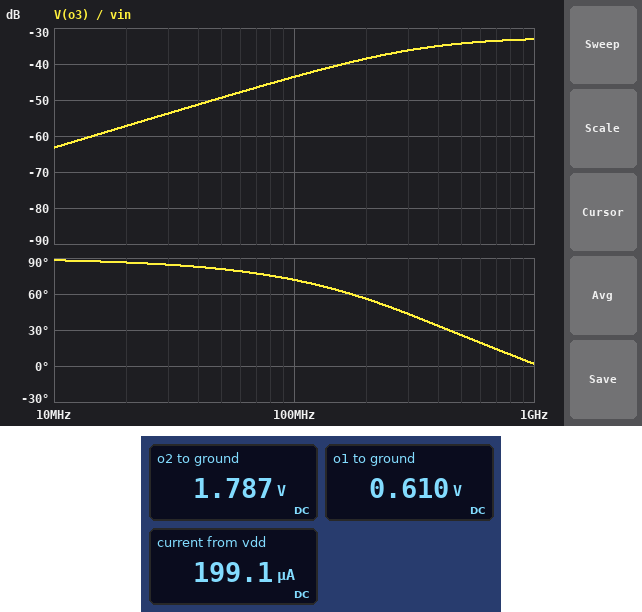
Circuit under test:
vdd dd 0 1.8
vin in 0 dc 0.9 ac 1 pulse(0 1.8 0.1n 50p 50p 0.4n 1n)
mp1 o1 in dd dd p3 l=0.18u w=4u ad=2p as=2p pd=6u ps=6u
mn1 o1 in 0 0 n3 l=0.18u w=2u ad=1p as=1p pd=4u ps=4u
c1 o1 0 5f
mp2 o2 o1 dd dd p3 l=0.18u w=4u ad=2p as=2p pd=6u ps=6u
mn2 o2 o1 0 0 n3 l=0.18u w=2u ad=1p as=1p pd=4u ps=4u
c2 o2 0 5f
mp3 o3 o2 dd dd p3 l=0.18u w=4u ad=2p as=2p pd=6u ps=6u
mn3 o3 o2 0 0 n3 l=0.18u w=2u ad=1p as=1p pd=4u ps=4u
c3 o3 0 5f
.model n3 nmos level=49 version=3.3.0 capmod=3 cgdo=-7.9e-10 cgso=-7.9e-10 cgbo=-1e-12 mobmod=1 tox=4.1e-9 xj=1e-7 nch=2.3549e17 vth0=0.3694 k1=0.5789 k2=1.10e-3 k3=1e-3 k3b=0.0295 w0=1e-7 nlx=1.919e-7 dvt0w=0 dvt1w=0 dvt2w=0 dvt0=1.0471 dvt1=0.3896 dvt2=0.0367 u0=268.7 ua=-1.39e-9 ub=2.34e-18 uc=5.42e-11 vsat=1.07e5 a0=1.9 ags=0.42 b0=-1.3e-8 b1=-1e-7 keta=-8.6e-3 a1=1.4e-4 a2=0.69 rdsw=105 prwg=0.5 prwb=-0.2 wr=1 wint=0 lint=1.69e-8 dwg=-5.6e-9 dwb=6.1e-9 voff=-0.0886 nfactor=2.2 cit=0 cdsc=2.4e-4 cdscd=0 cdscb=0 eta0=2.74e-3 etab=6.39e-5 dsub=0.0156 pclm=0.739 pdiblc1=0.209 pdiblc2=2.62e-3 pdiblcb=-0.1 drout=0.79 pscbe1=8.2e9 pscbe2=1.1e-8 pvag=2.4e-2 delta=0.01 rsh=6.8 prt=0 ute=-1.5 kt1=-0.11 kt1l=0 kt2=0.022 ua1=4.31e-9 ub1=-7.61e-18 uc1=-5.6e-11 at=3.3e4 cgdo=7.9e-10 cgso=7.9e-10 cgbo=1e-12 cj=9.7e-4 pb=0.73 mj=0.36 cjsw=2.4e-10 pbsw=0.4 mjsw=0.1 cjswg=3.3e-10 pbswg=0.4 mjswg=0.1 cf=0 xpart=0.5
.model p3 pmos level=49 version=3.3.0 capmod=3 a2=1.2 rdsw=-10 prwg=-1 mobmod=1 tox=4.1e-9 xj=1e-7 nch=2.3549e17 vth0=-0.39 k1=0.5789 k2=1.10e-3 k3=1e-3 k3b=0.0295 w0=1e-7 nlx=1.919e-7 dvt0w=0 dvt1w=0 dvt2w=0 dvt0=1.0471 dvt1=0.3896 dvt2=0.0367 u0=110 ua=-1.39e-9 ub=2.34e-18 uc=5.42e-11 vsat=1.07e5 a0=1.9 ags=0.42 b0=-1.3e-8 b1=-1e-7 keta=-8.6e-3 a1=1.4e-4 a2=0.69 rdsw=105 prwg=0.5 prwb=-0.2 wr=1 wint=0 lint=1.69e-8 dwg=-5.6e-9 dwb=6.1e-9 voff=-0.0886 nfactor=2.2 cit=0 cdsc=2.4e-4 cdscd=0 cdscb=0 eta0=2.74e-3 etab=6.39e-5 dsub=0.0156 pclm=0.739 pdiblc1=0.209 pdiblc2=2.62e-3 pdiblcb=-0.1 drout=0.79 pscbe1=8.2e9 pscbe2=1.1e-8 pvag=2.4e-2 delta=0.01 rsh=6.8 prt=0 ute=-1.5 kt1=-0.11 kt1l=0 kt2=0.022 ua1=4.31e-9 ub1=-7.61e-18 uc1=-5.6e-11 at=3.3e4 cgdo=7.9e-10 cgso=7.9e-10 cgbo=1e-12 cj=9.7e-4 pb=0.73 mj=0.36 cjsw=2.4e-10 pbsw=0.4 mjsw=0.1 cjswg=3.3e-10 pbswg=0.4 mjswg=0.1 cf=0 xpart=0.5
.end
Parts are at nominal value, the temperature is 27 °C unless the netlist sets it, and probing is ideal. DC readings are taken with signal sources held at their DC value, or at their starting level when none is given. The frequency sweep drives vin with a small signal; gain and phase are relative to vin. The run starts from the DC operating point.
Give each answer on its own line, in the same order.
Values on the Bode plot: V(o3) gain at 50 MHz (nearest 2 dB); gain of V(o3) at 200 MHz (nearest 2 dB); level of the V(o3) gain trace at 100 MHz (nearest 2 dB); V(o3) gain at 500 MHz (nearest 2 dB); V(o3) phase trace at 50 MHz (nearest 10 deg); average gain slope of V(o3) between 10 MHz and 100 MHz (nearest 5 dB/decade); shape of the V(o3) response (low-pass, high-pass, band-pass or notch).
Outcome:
-50 dB
-38 dB
-44 dB
-34 dB
80 deg
20 dB/decade
high-pass
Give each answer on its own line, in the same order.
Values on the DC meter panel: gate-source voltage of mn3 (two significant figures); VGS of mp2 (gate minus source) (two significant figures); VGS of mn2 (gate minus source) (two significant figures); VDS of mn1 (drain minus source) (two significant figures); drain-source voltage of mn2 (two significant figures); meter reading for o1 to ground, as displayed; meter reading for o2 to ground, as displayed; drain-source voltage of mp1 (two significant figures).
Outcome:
1.8 V
-1.2 V
610 mV
610 mV
1.8 V
0.610 V
1.787 V
-1.2 V
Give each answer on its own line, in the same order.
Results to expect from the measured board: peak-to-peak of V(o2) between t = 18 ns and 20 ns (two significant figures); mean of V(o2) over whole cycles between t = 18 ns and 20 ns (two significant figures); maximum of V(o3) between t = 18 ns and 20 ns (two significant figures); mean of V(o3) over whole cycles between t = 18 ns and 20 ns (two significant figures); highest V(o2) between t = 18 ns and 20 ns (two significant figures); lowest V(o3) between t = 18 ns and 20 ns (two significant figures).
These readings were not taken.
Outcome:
2.0 V
810 mV
1.9 V
1.0 V
1.9 V
-84 mV
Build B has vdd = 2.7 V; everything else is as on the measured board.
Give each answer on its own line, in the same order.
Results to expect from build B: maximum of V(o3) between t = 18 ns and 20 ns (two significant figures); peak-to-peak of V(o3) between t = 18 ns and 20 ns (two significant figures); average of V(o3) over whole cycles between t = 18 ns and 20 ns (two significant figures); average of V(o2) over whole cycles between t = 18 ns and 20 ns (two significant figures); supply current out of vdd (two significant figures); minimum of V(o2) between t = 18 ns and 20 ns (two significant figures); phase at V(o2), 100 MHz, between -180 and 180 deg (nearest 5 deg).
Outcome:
2.8 V
2.9 V
1.6 V
1.1 V
240 µA
-55 mV
-90 deg
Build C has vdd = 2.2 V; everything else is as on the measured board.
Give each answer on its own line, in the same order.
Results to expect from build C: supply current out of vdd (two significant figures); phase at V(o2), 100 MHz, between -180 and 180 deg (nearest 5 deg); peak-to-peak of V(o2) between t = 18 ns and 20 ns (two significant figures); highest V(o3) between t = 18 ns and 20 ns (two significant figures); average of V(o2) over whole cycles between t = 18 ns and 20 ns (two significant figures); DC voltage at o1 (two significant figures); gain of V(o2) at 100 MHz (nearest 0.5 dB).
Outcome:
220 µA
-90 deg
2.4 V
2.3 V
950 mV
2.1 V
-60.5 dB
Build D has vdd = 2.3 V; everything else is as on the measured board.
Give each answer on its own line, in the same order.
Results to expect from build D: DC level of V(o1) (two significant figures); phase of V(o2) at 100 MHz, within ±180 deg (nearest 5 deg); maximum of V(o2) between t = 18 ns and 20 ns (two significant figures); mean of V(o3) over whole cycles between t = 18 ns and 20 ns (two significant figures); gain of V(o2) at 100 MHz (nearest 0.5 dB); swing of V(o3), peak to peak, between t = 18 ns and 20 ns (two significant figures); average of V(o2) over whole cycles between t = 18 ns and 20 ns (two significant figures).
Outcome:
2.2 V
-90 deg
2.4 V
1.3 V
-62.5 dB
2.5 V
990 mV
